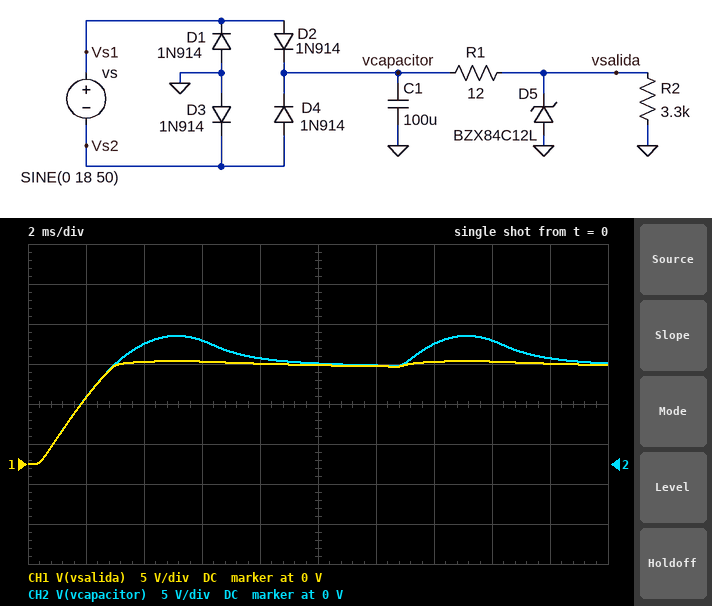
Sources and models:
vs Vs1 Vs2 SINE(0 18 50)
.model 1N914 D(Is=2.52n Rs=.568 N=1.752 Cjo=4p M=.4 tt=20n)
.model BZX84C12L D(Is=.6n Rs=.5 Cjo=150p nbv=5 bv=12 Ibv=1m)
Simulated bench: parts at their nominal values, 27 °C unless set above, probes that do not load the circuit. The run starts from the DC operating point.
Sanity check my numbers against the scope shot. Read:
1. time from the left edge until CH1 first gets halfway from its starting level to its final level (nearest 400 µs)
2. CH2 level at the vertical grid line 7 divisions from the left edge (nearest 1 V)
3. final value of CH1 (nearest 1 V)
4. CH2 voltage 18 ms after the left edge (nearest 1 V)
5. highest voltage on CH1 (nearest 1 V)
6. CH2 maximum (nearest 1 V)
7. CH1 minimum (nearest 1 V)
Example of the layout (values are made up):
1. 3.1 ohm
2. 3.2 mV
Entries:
1. 1.6 ms
2. 15 V
3. 12 V
4. 13 V
5. 13 V
6. 16 V
7. 0 V
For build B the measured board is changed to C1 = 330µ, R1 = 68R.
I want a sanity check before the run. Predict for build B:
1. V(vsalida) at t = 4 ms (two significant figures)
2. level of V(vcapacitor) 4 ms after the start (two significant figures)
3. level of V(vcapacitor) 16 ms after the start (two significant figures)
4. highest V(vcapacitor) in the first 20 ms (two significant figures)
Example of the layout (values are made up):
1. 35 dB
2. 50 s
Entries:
1. 12 V
2. 14 V
3. 16 V
4. 16 V
